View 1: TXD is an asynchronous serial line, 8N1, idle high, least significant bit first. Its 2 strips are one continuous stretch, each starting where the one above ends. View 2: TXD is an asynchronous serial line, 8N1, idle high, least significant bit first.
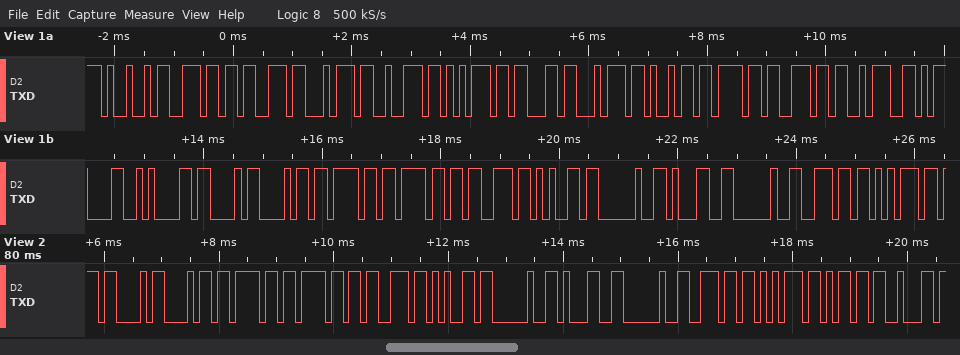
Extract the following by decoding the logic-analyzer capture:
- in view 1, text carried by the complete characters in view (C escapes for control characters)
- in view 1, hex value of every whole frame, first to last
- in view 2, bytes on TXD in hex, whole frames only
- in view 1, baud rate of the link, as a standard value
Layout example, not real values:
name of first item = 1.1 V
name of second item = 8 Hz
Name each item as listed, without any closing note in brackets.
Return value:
in view 1, text carried by the complete characters in view = "Instruction:\r\nChoose 1 nu"
in view 1, hex value of every whole frame, first to last = 49 6E 73 74 72 75 63 74 69 6F 6E 3A 0D 0A 43 68 6F 6F 73 65 20 31 20 6E 75
in view 2, bytes on TXD in hex, whole frames only = 0x43 0x68 0x6F 0x6F 0x73 0x65 0x20 0x31 0x20 0x6E 0x75 0x6D 0x62
in view 1, baud rate of the link, as a standard value = 9600 baud
